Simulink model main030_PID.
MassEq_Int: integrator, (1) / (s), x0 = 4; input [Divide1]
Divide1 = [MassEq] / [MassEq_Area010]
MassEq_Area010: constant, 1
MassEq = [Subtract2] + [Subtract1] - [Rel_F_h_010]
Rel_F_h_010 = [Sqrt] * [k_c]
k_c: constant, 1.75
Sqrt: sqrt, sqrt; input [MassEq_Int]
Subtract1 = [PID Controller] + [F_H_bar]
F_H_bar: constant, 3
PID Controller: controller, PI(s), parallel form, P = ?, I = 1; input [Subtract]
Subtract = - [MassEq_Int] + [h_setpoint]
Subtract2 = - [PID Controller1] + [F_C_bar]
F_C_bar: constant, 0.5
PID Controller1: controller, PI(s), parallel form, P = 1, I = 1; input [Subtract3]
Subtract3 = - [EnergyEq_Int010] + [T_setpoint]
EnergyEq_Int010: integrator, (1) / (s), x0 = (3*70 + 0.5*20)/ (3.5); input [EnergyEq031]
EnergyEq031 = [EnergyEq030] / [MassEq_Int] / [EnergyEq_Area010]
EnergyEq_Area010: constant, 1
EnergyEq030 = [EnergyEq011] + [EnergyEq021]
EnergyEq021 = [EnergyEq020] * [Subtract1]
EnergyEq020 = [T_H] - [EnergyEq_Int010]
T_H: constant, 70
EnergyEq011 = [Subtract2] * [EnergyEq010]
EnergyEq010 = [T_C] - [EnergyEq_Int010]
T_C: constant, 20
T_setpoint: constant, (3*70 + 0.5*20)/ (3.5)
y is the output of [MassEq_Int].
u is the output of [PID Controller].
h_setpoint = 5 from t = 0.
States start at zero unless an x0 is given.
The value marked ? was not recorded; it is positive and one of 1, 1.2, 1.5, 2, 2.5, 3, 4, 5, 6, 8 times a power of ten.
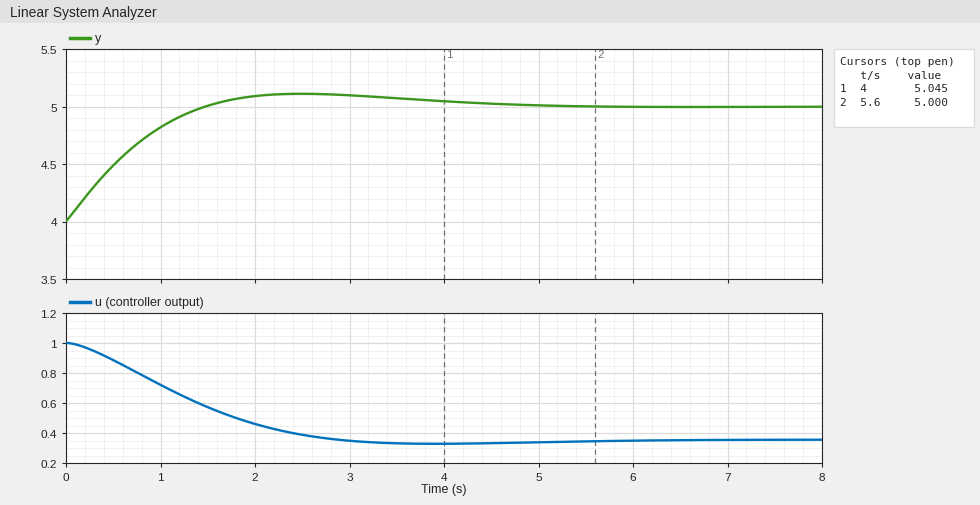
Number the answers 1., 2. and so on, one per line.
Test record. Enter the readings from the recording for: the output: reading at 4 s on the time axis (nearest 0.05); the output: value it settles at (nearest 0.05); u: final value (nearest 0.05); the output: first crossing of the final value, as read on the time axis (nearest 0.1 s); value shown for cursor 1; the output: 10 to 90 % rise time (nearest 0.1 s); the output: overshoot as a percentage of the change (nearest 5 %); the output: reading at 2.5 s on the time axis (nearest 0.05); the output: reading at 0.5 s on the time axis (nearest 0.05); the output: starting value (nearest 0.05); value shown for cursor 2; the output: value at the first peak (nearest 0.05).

1. 5.05
2. 5.00
3. 0.35
4. 1.5 s
5. 5.045
6. 1.1 s
7. 10 %
8. 5.10
9. 4.50
10. 4.00
11. 5.000
12. 5.10
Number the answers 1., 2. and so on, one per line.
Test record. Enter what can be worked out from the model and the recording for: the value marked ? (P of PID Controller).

1. 1
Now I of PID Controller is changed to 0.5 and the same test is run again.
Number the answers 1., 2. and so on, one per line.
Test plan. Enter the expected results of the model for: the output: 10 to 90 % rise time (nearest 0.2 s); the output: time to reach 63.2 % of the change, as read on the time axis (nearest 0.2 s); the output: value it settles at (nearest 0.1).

1. 1.6 s
2. 0.8 s
3. 5.0
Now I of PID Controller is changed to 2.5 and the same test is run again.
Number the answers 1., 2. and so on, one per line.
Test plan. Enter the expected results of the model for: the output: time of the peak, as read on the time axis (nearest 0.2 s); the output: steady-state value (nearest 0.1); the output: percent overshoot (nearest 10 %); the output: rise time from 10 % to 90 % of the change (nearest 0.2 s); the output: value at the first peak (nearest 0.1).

1. 1.6 s
2. 5.0
3. 30 %
4. 0.6 s
5. 5.3
